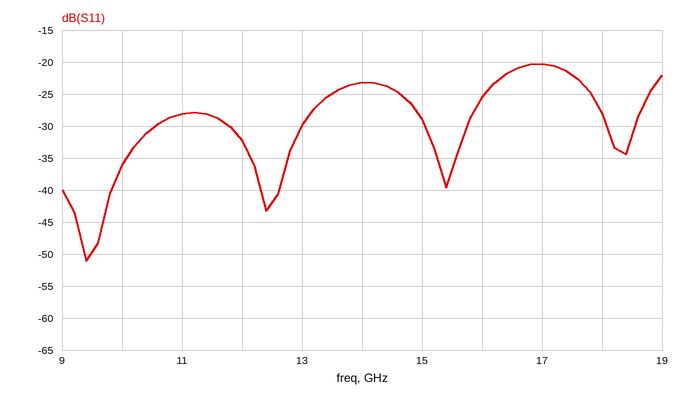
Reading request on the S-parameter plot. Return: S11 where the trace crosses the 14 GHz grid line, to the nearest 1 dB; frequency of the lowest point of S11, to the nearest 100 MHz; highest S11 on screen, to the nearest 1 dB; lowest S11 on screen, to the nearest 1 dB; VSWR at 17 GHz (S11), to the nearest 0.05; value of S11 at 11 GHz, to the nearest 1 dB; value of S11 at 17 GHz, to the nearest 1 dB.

-23 dB
9.4 GHz
-20 dB
-51 dB
1.20
-28 dB
-20 dB
